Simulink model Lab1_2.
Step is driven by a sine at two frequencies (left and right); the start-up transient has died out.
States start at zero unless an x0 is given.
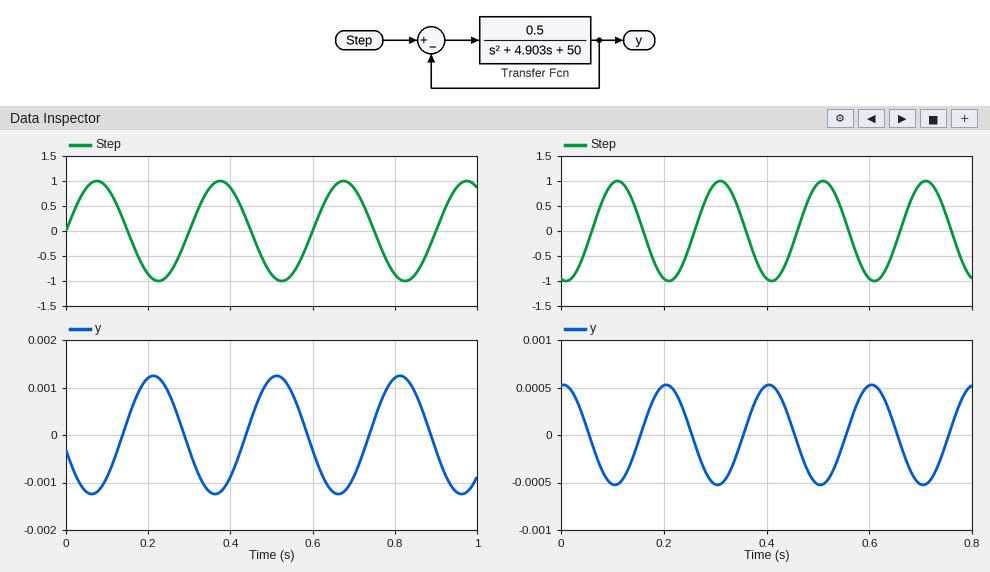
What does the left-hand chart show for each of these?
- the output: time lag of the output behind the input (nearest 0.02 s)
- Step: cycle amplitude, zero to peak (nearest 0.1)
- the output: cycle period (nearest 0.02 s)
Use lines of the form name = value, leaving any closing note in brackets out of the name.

the output: time lag of the output behind the input = 0.14 s
Step: cycle amplitude, zero to peak = 1.0
the output: cycle period = 0.30 s
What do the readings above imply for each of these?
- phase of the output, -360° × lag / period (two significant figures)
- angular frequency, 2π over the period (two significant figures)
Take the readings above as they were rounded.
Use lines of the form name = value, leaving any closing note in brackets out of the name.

phase of the output, -360° × lag / period = -170°
angular frequency, 2π over the period = 21 rad/s
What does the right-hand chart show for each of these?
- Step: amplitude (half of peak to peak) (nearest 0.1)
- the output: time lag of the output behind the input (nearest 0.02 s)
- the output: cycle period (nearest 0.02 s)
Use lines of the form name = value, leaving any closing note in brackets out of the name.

Step: amplitude (half of peak to peak) = 1.0
the output: time lag of the output behind the input = 0.10 s
the output: cycle period = 0.20 s
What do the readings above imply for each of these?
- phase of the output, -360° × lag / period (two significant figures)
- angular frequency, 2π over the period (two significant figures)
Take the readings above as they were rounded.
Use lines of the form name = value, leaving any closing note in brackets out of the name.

phase of the output, -360° × lag / period = -180°
angular frequency, 2π over the period = 31 rad/s
